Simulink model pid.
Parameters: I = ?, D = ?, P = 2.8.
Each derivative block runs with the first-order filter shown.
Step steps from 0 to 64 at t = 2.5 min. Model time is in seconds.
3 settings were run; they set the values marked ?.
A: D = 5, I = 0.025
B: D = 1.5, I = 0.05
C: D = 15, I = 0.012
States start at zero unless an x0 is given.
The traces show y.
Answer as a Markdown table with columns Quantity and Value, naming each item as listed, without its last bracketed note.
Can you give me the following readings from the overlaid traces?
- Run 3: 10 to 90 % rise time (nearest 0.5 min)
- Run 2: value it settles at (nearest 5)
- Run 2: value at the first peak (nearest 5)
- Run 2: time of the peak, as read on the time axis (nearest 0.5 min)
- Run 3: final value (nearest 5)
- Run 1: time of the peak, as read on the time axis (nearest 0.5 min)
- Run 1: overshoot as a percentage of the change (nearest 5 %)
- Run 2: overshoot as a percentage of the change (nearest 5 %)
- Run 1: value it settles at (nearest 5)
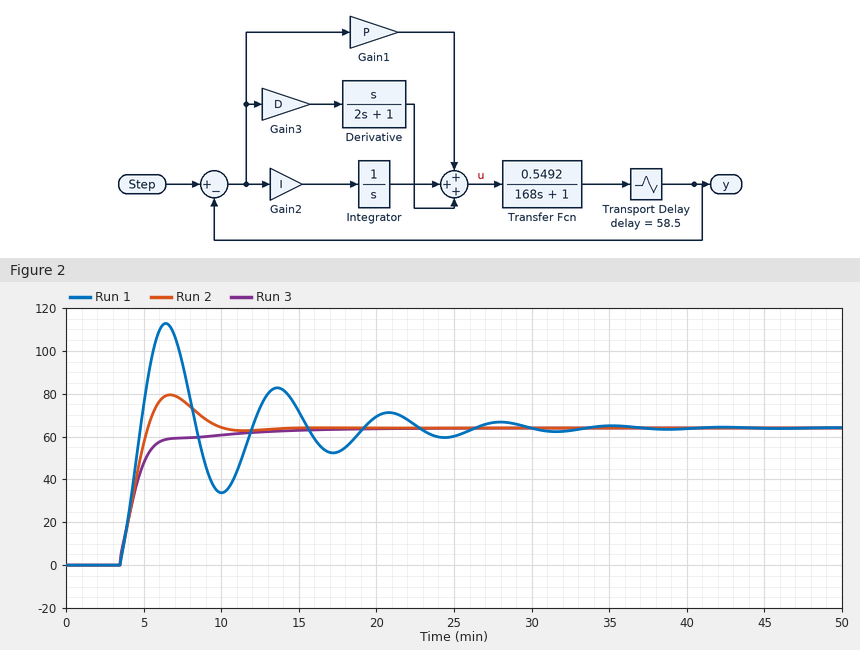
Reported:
| Quantity | Value |
|---|---|
| Run 3: 10 to 90 % rise time | 2.5 min |
| Run 2: value it settles at | 65 |
| Run 2: value at the first peak | 80 |
| Run 2: time of the peak, as read on the time axis | 6.5 min |
| Run 3: final value | 65 |
| Run 1: time of the peak, as read on the time axis | 6.5 min |
| Run 1: overshoot as a percentage of the change | 75 % |
| Run 2: overshoot as a percentage of the change | 25 % |
| Run 1: value it settles at | 65 |
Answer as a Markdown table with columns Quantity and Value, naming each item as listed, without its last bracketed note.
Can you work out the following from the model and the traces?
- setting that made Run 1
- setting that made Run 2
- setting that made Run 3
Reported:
| Quantity | Value |
|---|---|
| setting that made Run 1 | B |
| setting that made Run 2 | A |
| setting that made Run 3 | C |
